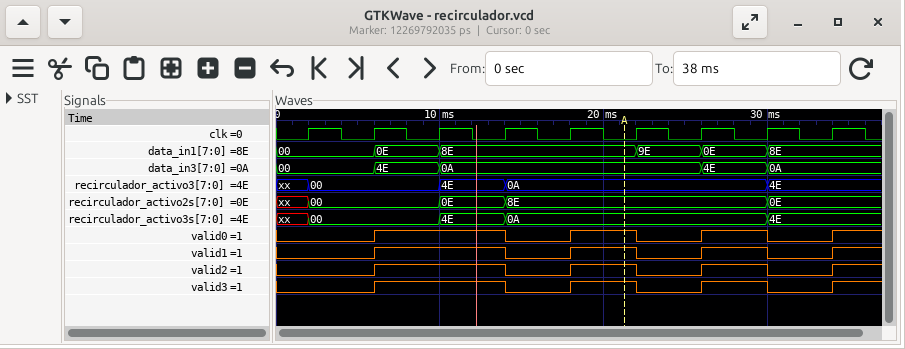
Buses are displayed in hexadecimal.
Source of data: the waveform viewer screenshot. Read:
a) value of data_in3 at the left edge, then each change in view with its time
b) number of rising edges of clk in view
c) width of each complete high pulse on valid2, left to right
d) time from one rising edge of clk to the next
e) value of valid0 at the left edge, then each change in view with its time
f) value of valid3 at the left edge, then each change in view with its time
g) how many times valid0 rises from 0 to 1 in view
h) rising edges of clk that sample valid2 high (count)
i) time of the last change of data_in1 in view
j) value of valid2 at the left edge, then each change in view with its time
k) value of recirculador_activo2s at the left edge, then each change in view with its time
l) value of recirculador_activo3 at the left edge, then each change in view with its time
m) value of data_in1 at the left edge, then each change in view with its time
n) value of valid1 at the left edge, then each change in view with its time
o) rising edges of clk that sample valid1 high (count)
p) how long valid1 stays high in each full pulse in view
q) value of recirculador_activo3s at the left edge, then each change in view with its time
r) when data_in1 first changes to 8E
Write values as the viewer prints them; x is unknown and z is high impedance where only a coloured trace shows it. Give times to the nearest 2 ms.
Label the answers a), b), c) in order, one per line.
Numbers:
a) 00, 4E at 6 ms, 0A at 10 ms, 4E at 26 ms, 0A at 30 ms
b) 9
c) 8 ms, 4 ms, 4 ms
d) 4 ms
e) 0, 1 at 6 ms, 0 at 14 ms, 1 at 18 ms, 0 at 22 ms, 1 at 26 ms, 0 at 30 ms, 1 at 34 ms
f) 0, 1 at 6 ms, 0 at 14 ms, 1 at 18 ms, 0 at 22 ms, 1 at 26 ms, 0 at 30 ms, 1 at 34 ms
g) 4
h) 4
i) 30 ms
j) 0, 1 at 6 ms, 0 at 14 ms, 1 at 18 ms, 0 at 22 ms, 1 at 26 ms, 0 at 30 ms, 1 at 34 ms
k) xx, 00 at 2 ms, 0E at 10 ms, 8E at 14 ms, 0E at 30 ms
l) xx, 00 at 2 ms, 4E at 10 ms, 0A at 14 ms, 4E at 30 ms
m) 00, 0E at 6 ms, 8E at 10 ms, 9E at 22 ms, 0E at 26 ms, 8E at 30 ms
n) 0, 1 at 6 ms, 0 at 14 ms, 1 at 18 ms, 0 at 22 ms, 1 at 26 ms, 0 at 30 ms, 1 at 34 ms
o) 4
p) 8 ms, 4 ms, 4 ms
q) xx, 00 at 2 ms, 4E at 10 ms, 0A at 14 ms, 4E at 30 ms
r) 10 ms
